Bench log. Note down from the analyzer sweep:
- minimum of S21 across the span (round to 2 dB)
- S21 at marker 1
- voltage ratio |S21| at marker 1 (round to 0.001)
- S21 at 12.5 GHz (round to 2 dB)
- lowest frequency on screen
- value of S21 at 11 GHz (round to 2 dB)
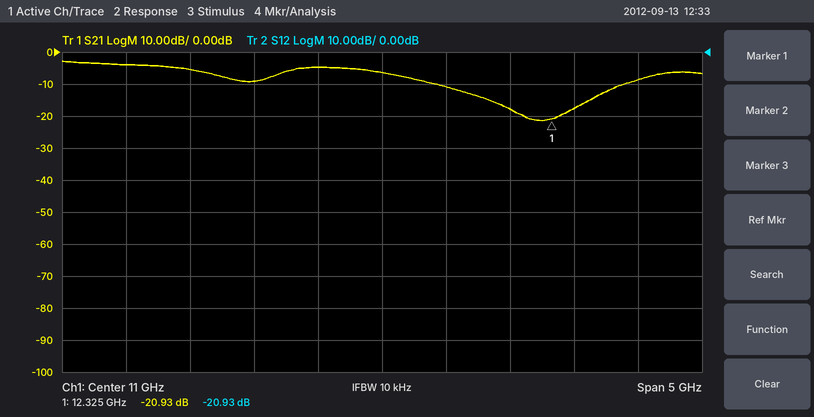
-22 dB
-20.93 dB
0.090
-18 dB
8.5 GHz
-6 dB
